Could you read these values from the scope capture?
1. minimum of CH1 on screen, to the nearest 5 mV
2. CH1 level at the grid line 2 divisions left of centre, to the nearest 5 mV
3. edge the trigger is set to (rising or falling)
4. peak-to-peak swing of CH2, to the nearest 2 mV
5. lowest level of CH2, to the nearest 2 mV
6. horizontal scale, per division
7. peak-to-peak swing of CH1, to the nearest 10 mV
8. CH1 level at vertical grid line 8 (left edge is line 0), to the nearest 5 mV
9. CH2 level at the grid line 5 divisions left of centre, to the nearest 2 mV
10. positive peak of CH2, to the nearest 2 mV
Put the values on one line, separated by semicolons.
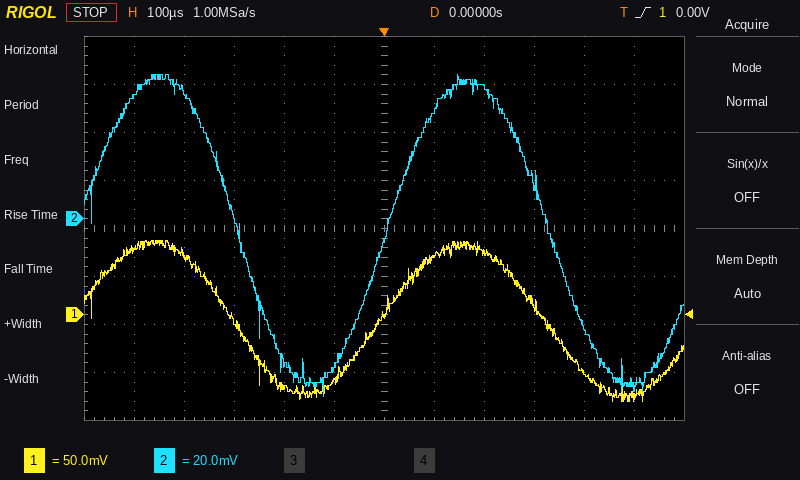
-90 mV; -75 mV; rising; 134 mV; -74 mV; 100 µs; 170 mV; 65 mV; 52 mV; 60 mV
